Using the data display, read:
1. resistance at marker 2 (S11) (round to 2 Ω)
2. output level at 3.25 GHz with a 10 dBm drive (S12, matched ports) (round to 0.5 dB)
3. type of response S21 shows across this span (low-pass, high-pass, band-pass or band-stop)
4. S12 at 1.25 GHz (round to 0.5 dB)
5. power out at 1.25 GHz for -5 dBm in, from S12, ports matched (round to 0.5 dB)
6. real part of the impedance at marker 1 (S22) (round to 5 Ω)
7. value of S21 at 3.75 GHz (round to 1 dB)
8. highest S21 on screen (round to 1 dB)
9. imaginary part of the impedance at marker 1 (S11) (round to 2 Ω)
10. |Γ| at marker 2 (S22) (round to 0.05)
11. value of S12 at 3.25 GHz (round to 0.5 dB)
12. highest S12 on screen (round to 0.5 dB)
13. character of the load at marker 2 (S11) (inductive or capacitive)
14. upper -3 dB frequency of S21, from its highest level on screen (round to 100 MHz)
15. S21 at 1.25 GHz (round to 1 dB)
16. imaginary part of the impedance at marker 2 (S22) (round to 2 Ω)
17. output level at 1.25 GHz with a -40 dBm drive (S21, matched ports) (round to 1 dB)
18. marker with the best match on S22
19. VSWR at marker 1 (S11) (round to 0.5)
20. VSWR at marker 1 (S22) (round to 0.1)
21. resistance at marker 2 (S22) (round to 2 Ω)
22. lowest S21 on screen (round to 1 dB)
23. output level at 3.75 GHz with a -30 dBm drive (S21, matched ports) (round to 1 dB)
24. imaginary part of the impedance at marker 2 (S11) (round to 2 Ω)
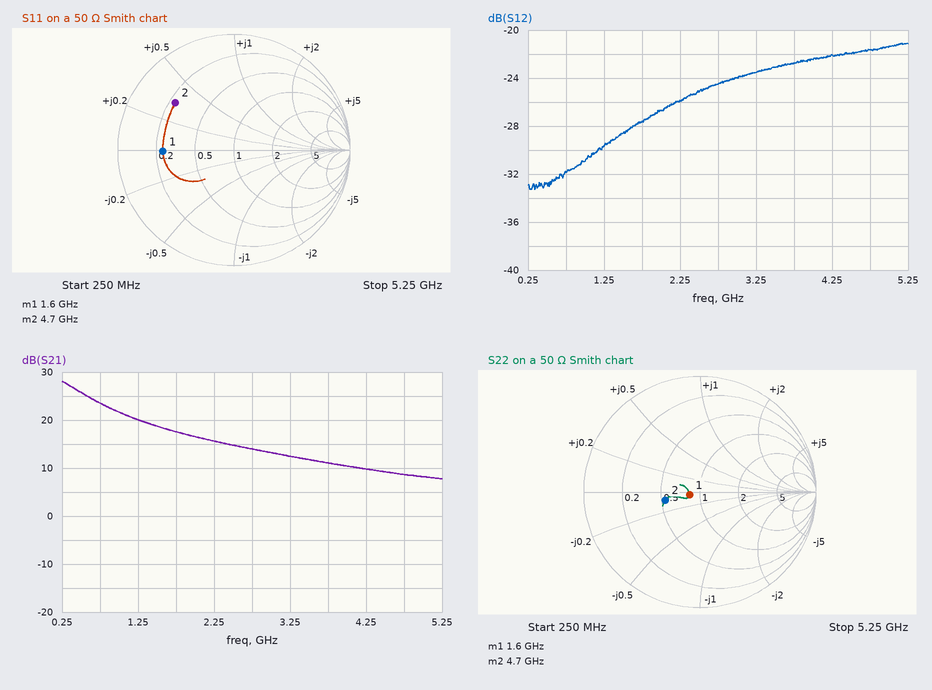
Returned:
12 Ω
-13.5 dBm
low-pass
-29.5 dB
-34.5 dBm
40 Ω
11 dB
28 dB
0 Ω
0.30
-23.5 dB
-21.0 dB
inductive
600 MHz
20 dB
-4 Ω
-20 dBm
marker 1
4.0
1.2
26 Ω
8 dB
-19 dBm
+16 Ω
